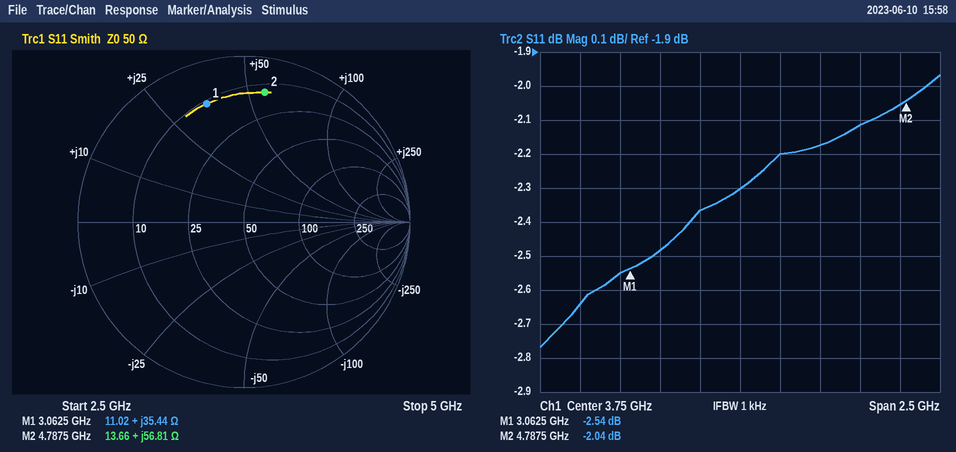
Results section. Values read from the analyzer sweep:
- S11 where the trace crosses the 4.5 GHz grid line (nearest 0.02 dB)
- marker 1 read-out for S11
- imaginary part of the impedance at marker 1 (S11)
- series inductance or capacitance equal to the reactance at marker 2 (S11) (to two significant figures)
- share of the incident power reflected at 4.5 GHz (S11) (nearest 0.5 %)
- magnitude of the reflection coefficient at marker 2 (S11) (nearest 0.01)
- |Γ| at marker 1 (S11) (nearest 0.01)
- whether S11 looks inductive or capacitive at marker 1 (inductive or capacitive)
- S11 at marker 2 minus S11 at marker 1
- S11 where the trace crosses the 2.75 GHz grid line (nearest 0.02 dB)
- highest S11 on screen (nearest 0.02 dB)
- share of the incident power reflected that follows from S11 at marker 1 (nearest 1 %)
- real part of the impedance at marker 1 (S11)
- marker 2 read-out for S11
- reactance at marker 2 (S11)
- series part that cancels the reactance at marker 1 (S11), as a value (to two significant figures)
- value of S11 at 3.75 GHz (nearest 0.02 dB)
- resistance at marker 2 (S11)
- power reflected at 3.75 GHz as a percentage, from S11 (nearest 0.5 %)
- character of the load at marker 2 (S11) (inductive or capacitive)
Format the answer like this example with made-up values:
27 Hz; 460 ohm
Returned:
-2.12 dB; -2.54 dB; +35.44 Ω; 1.9 nH; 61.5 %; 0.79; 0.75; inductive; 0.50 dB; -2.64 dB; -1.96 dB; 56 %; 11.02 Ω; -2.04 dB; +56.81 Ω; 1.5 pF; -2.30 dB; 13.66 Ω; 59.0 %; inductive
